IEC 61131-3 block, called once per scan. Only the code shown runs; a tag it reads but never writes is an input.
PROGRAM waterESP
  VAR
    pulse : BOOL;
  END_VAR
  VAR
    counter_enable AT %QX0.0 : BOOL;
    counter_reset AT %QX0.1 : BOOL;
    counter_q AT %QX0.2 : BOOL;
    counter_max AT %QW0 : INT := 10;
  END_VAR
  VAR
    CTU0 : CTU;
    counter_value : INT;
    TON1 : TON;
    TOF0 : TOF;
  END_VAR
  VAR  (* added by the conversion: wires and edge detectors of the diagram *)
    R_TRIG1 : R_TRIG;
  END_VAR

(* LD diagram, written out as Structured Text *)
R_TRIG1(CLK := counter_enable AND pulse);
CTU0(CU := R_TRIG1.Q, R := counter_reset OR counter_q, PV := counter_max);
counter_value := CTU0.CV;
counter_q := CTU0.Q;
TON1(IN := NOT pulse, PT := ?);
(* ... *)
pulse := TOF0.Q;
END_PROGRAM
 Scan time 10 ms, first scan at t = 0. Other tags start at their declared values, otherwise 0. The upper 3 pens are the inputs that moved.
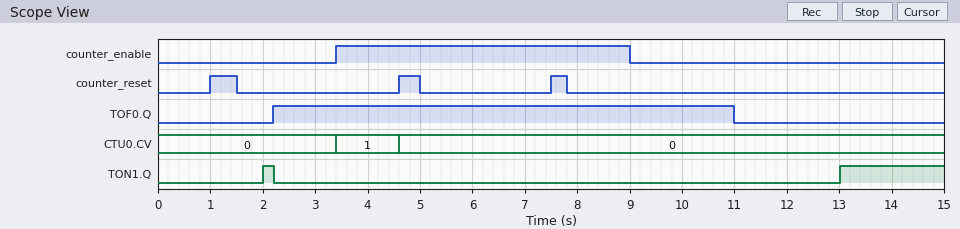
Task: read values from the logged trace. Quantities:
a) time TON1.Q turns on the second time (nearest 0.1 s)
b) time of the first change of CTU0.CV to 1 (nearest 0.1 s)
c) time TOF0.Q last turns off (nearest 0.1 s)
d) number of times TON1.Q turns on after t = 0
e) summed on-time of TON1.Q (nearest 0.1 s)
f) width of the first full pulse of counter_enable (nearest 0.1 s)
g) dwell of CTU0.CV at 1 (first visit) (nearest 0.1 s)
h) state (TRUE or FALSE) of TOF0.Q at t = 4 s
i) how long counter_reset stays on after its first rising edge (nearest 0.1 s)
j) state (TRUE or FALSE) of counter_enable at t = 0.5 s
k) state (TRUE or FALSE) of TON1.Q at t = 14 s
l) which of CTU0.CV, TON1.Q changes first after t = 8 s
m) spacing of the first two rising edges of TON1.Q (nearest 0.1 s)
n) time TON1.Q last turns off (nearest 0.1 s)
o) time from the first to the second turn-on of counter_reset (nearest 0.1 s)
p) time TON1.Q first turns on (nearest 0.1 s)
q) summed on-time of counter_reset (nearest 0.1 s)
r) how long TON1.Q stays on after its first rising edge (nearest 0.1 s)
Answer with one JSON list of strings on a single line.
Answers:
["13.0 s", "3.4 s", "11.0 s", "2", "2.2 s", "5.6 s", "1.2 s", "TRUE", "0.5 s", "FALSE", "TRUE", "TON1.Q", "11.0 s", "2.2 s", "3.6 s", "2.0 s", "1.2 s", "0.2 s"]
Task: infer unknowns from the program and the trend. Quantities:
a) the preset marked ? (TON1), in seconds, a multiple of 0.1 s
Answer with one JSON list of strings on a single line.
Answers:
["2.0 s"]
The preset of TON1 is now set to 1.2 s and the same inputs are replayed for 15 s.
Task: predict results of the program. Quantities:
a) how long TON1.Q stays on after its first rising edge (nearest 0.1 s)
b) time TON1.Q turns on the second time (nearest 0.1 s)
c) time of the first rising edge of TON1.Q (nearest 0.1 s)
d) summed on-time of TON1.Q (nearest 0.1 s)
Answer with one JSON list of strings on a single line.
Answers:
["1.0 s", "12.2 s", "1.2 s", "3.8 s"]
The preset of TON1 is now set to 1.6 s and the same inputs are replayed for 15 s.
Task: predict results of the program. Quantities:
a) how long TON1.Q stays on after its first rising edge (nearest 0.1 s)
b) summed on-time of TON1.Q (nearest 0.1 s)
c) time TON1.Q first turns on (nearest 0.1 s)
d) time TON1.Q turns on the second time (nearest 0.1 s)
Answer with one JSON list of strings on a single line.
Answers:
["0.6 s", "3.0 s", "1.6 s", "12.6 s"]
